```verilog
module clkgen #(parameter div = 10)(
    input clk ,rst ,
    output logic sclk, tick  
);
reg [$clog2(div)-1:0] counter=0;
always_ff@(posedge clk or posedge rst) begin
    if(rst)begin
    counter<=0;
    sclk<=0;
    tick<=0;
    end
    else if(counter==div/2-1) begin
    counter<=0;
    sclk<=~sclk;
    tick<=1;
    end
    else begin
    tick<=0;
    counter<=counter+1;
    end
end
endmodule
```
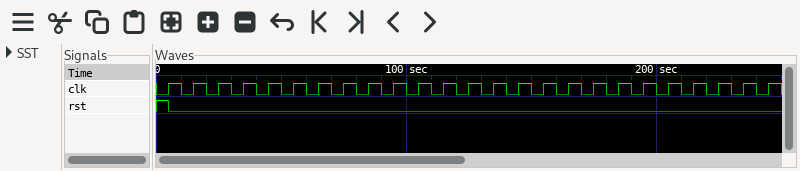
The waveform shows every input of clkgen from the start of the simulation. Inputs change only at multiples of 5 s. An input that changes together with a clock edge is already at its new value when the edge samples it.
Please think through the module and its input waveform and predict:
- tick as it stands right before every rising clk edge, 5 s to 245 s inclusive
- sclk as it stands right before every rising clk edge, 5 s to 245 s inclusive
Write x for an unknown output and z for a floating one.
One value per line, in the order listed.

0 0 0 0 0 1 0 0 0 0 1 0 0 0 0 1 0 0 0 0 1 0 0 0 0
0 0 0 0 0 1 1 1 1 1 0 0 0 0 0 1 1 1 1 1 0 0 0 0 0
